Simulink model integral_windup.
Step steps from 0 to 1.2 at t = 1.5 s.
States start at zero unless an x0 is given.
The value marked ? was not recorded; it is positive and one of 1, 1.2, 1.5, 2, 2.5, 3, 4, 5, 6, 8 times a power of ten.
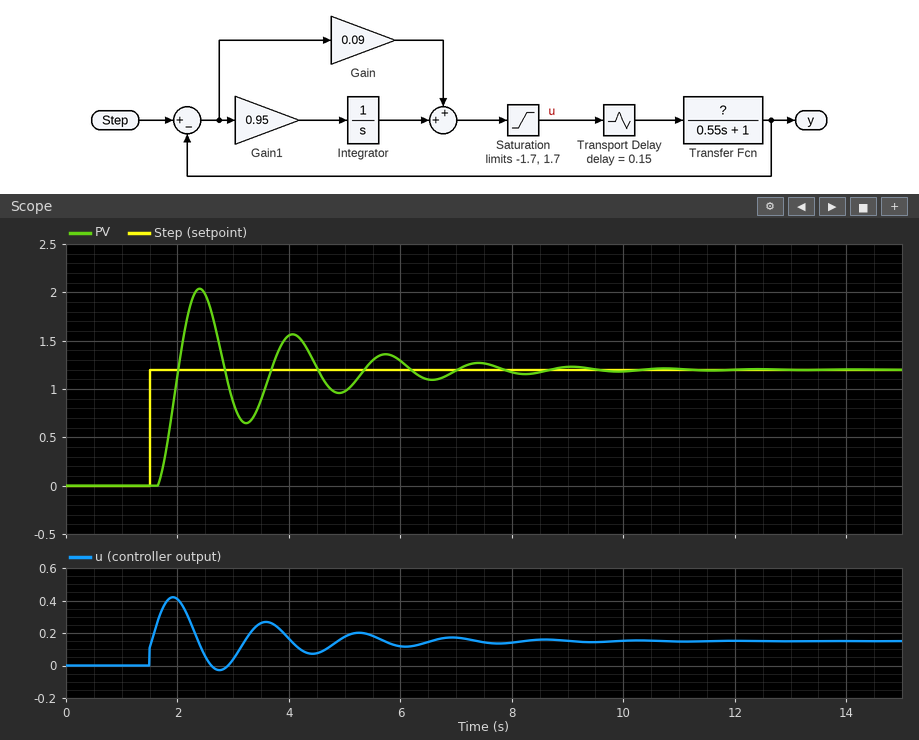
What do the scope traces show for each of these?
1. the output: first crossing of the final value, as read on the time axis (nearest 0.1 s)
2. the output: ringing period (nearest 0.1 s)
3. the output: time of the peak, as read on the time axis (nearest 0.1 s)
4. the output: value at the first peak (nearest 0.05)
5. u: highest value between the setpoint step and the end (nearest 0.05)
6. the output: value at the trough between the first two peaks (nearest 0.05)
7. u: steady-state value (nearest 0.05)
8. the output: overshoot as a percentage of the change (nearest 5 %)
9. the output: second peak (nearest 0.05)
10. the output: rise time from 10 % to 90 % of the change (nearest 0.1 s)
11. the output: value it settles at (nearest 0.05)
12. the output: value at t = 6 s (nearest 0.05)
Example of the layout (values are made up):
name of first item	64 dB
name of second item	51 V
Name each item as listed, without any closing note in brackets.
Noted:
the output: first crossing of the final value, as read on the time axis	2.0 s
the output: ringing period	1.7 s
the output: time of the peak, as read on the time axis	2.4 s
the output: value at the first peak	2.05
u: highest value between the setpoint step and the end	0.40
the output: value at the trough between the first two peaks	0.65
u: steady-state value	0.15
the output: overshoot as a percentage of the change	70 %
the output: second peak	1.55
the output: rise time from 10 % to 90 % of the change	0.3 s
the output: value it settles at	1.20
the output: value at t = 6 s	1.30
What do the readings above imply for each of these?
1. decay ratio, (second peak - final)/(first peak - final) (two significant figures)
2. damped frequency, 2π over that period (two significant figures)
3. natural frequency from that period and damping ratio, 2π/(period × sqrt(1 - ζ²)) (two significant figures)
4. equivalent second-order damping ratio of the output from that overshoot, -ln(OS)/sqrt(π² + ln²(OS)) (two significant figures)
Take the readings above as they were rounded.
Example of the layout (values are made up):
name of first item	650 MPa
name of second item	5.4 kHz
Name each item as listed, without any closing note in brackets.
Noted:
decay ratio, (second peak - final)/(first peak - final)	0.41
damped frequency, 2π over that period	3.7 rad/s
natural frequency from that period and damping ratio, 2π/(period × sqrt(1 - ζ²))	3.7 rad/s
equivalent second-order damping ratio of the output from that overshoot, -ln(OS)/sqrt(π² + ln²(OS))	0.11
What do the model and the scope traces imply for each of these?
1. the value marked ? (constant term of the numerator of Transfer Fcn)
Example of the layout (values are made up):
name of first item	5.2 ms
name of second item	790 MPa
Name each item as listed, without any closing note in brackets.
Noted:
the value marked ?	8
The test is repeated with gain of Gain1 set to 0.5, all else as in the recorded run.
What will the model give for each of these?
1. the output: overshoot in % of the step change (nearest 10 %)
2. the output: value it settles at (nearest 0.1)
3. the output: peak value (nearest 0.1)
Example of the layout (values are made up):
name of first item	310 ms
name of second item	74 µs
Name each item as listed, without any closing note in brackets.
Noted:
the output: overshoot in % of the step change	30 %
the output: value it settles at	1.2
the output: peak value	1.6
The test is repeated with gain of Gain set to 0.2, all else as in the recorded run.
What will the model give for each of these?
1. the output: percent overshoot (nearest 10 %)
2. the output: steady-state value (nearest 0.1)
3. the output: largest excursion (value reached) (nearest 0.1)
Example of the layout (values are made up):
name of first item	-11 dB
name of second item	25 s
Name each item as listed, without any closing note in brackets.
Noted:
the output: percent overshoot	50 %
the output: steady-state value	1.2
the output: largest excursion (value reached)	1.8
